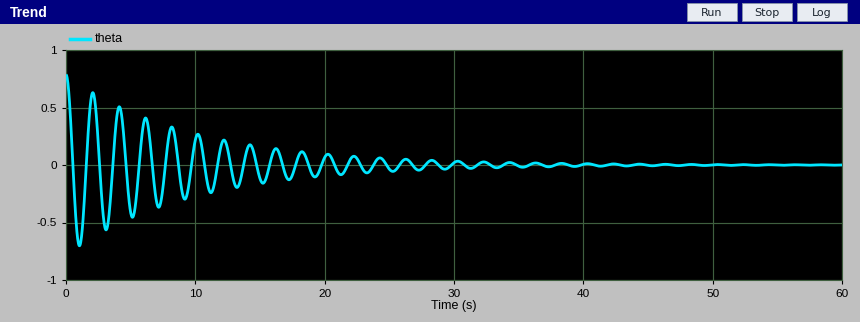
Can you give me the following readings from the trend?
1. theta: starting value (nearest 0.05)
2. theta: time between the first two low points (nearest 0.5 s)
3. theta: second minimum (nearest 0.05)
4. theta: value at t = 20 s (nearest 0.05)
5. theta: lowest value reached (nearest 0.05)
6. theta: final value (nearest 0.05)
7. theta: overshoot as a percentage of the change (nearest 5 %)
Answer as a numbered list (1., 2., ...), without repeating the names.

1. 0.80
2. 2.0 s
3. -0.55
4. 0.05
5. -0.70
6. 0.00
7. 90 %
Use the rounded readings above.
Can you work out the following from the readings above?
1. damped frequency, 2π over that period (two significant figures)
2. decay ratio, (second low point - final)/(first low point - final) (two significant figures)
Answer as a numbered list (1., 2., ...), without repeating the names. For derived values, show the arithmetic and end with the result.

1. 2π / 2 = 3.1 rad/s
2. (-0.55 - 0) / (-0.7 - 0) = 0.79
